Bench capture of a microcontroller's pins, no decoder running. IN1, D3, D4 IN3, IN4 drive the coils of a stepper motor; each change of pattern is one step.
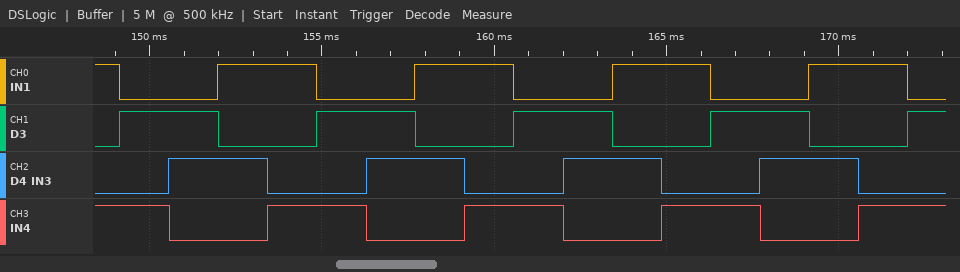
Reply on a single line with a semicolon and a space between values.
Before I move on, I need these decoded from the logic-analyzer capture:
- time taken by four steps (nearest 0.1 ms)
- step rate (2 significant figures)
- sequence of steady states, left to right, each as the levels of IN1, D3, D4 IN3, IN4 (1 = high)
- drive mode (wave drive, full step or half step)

5.7 ms; 700 steps/s; 1001 0101 0110 1010 1001 0101 0110 1010 1001 0101 0110 1010 1001 0101 0110 1010 1001 0101; full step
